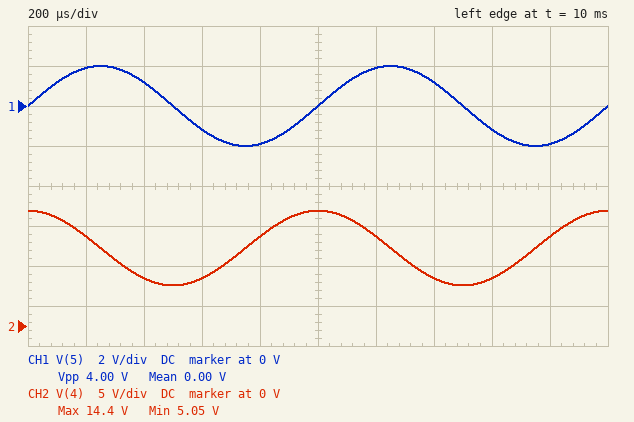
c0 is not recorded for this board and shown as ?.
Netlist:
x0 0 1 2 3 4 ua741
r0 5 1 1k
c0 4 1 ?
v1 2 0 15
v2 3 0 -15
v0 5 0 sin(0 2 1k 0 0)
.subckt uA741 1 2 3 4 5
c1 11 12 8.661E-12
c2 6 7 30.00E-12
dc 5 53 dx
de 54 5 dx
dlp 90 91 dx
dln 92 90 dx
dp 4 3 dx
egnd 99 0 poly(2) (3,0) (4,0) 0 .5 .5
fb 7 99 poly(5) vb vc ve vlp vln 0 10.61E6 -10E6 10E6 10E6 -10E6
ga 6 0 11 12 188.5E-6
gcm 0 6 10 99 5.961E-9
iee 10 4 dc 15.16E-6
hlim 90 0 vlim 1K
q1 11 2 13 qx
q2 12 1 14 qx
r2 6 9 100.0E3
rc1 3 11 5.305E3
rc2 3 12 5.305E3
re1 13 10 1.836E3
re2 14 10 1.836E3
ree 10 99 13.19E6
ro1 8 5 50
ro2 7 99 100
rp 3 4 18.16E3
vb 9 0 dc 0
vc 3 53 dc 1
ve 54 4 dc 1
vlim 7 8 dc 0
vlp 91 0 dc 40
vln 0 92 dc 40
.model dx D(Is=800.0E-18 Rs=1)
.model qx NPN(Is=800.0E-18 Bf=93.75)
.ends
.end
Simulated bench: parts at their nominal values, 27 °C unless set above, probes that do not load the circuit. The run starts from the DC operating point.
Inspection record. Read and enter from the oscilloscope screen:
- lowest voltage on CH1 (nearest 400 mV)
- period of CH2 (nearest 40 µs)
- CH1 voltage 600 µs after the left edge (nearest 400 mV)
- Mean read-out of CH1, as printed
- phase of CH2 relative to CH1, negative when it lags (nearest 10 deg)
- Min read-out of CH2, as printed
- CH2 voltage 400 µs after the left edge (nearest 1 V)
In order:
-2.0 V
1.00 ms
-1.2 V
0.00 V
90 deg
5.05 V
6 V
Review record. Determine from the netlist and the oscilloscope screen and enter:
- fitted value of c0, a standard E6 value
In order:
68 nF
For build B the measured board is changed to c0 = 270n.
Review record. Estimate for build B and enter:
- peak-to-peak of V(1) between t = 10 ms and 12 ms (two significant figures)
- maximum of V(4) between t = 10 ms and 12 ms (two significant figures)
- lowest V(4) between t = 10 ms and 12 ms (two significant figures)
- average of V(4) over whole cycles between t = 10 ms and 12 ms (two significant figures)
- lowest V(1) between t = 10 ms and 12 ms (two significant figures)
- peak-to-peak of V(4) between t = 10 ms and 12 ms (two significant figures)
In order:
2.4 mV
14 V
12 V
13 V
-1.2 mV
2.4 V
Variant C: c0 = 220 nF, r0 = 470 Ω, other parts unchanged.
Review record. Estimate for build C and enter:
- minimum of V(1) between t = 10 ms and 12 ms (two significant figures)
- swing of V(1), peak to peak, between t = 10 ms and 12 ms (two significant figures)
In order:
-3.1 mV
6.2 mV
